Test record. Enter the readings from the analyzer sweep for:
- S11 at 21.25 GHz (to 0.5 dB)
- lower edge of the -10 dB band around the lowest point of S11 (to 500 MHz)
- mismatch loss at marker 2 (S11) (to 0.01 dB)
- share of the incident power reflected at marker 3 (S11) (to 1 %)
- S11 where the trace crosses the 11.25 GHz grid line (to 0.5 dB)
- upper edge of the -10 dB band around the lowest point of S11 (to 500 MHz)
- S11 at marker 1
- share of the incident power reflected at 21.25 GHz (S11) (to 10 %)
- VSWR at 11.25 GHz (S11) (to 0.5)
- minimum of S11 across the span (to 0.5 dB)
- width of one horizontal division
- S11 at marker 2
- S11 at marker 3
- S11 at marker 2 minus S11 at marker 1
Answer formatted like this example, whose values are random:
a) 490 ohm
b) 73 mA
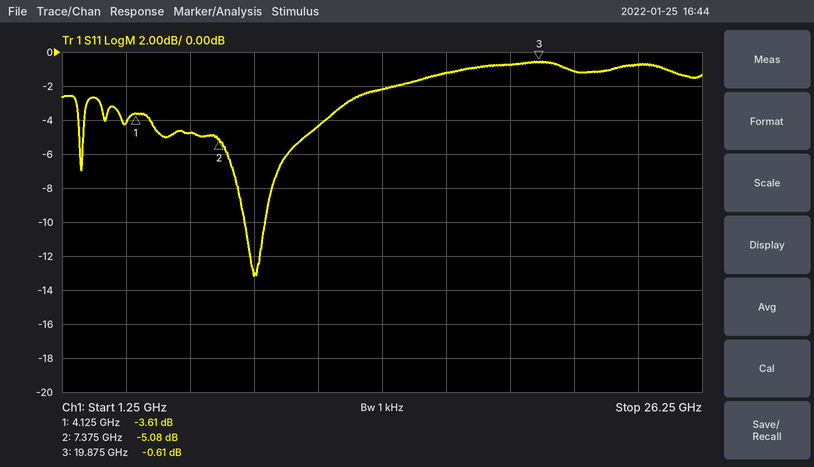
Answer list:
a) -1.0 dB
b) 8.5 GHz
c) 1.61 dB
d) 87 %
e) -4.5 dB
f) 9.0 GHz
g) -3.61 dB
h) 80 %
i) 4.0
j) -13.0 dB
k) 2.5 GHz
l) -5.08 dB
m) -0.61 dB
n) -1.47 dB
